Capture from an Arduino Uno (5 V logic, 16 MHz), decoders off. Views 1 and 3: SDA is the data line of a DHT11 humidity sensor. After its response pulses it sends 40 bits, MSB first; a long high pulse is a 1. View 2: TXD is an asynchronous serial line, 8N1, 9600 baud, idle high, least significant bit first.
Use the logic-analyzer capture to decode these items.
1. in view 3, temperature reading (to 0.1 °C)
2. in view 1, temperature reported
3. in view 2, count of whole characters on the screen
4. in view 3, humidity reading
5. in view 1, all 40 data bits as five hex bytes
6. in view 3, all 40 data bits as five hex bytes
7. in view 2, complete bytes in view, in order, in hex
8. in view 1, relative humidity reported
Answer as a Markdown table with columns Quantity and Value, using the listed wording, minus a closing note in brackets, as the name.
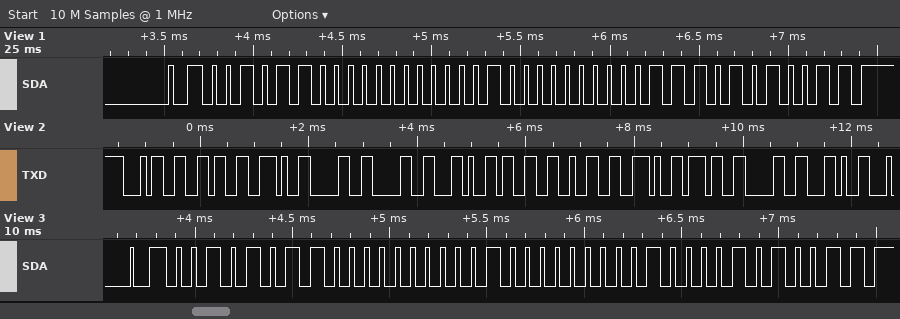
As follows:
| Quantity | Value |
|---|---|
| in view 3, temperature reading | 32.8 °C |
| in view 1, temperature reported | 32.7 °C |
| in view 2, count of whole characters on the screen | 12 |
| in view 3, humidity reading | 43 % |
| in view 1, all 40 data bits as five hex bytes | 2C 00 20 07 53 |
| in view 3, all 40 data bits as five hex bytes | 2B 00 20 08 53 |
| in view 2, complete bytes in view, in order, in hex | 34 36 2E 30 30 2C 33 32 2E 37 30 2C |
| in view 1, relative humidity reported | 44 % |
